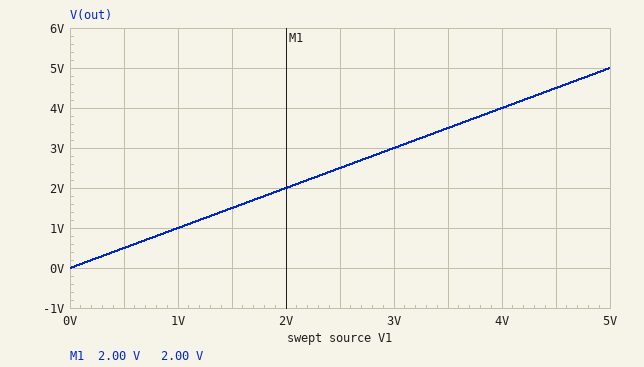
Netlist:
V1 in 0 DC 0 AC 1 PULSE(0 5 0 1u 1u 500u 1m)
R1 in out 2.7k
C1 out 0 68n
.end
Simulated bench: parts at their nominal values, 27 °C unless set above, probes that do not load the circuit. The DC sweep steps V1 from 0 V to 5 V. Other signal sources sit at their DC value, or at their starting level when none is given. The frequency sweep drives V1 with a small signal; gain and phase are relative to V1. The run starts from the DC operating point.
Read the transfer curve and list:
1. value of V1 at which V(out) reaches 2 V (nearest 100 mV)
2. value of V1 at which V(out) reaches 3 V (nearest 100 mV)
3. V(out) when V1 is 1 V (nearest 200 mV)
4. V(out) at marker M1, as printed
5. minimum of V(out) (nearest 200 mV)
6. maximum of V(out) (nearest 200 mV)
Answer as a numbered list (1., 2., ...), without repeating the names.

1. 2.0 V
2. 3.0 V
3. 1.0 V
4. 2.00 V
5. 0 V
6. 5.0 V
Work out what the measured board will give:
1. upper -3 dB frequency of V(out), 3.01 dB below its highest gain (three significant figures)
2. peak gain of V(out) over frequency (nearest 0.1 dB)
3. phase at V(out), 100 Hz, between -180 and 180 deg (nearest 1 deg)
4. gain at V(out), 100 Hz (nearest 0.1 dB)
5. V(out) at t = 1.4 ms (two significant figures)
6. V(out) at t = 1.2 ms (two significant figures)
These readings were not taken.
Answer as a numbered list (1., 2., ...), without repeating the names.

1. 867 Hz
2. 0 dB
3. -7 deg
4. -0.1 dB
5. 4.5 V
6. 3.4 V
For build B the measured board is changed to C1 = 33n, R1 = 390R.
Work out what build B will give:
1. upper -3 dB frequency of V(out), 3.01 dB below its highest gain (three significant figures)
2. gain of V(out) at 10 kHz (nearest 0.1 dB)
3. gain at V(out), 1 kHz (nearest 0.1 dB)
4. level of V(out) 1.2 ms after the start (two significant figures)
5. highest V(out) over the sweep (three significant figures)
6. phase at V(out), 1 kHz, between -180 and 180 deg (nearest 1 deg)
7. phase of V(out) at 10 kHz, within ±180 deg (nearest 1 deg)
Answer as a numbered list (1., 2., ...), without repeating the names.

1. 12.4 kHz
2. -2.2 dB
3. 0 dB
4. 5.0 V
5. 5.00 V
6. -5 deg
7. -39 deg
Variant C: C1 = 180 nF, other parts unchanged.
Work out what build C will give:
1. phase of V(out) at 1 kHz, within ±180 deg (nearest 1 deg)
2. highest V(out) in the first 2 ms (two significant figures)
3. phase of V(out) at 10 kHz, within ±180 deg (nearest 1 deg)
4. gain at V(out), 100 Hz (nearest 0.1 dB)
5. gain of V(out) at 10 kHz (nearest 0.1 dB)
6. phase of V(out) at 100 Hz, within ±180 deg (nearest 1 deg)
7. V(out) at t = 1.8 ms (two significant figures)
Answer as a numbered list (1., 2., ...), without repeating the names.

1. -72 deg
2. 3.6 V
3. -88 deg
4. -0.4 dB
5. -29.7 dB
6. -17 deg
7. 2.0 V
